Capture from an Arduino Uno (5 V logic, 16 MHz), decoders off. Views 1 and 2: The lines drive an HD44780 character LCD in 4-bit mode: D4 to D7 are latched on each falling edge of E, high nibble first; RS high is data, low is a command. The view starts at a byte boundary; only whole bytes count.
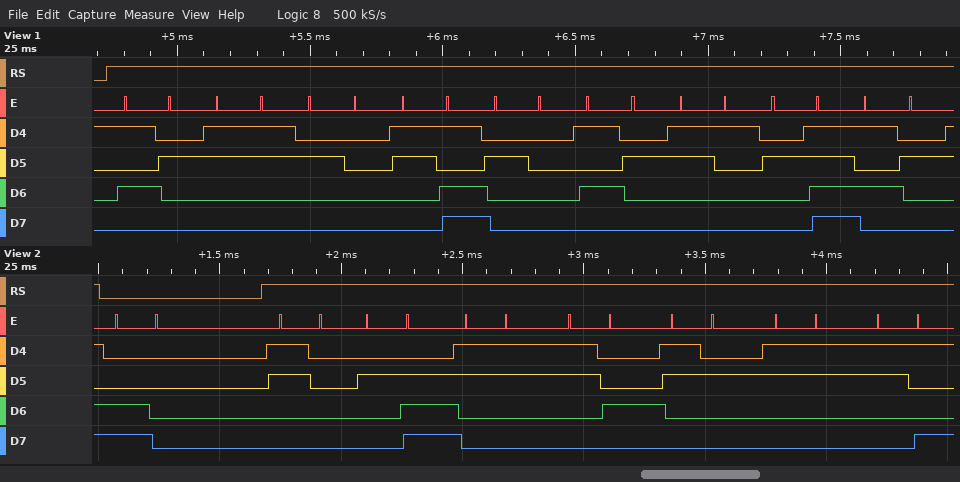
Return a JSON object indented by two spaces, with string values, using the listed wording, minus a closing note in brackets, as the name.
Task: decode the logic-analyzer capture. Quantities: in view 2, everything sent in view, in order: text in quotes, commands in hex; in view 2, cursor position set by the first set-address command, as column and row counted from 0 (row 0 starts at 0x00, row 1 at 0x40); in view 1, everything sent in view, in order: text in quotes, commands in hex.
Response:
{
  "in view 2, everything sent in view, in order: text in quotes, commands in hex": "0xC0 \"0.34239\"",
  "in view 2, cursor position set by the first set-address command, as column and row counted from 0": "column 0, row 1",
  "in view 1, everything sent in view, in order: text in quotes, commands in hex": "\"R3 = R1/R\""
}
